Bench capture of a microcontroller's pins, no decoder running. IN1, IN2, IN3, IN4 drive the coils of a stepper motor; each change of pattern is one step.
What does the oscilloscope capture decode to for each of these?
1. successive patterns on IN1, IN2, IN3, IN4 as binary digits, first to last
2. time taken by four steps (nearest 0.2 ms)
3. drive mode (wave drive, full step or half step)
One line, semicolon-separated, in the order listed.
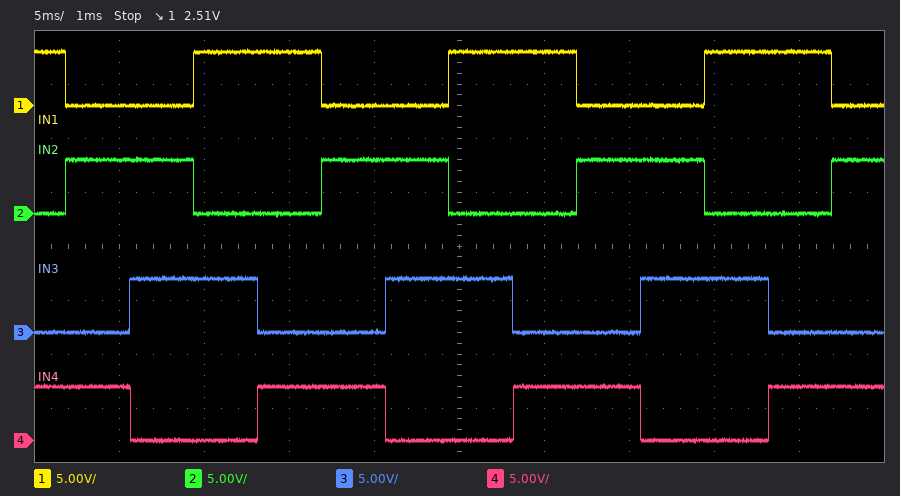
1001 0101 0110 1010 1001 0101 0110 1010 1001 0101 0110 1010 1001 0101; 15.0 ms; full step
